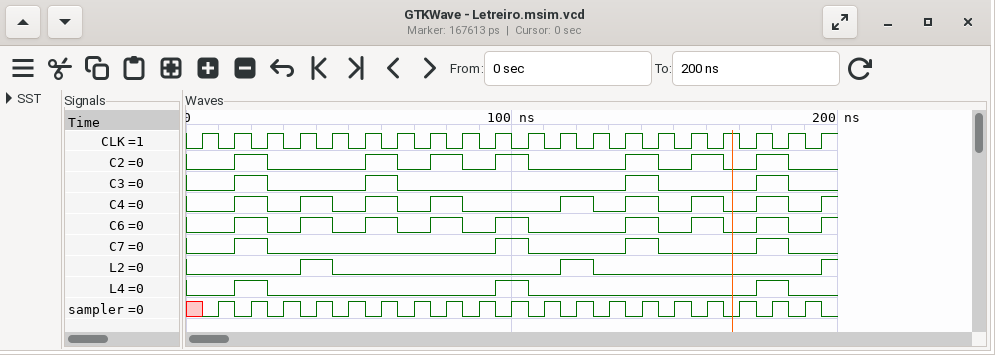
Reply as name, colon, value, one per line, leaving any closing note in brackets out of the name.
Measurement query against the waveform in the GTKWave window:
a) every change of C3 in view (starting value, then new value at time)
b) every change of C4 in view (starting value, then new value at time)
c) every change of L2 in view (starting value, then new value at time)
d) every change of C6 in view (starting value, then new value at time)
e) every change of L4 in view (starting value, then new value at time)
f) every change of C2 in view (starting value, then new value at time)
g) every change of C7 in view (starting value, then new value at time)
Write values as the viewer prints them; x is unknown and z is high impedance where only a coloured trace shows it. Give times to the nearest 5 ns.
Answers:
every change of C3 in view: 0, 1 at 15 ns, 0 at 25 ns, 1 at 55 ns, 0 at 65 ns, 1 at 135 ns, 0 at 145 ns, 1 at 175 ns, 0 at 185 ns
every change of C4 in view: 0, 1 at 15 ns, 0 at 25 ns, 1 at 35 ns, 0 at 45 ns, 1 at 55 ns, 0 at 65 ns, 1 at 75 ns, 0 at 85 ns, 1 at 115 ns, 0 at 125 ns, 1 at 135 ns, 0 at 145 ns, 1 at 155 ns, 0 at 165 ns, 1 at 175 ns, 0 at 185 ns, 1 at 195 ns
every change of L2 in view: 0, 1 at 35 ns, 0 at 45 ns, 1 at 115 ns, 0 at 125 ns, 1 at 195 ns
every change of C6 in view: 0, 1 at 15 ns, 0 at 25 ns, 1 at 35 ns, 0 at 45 ns, 1 at 55 ns, 0 at 65 ns, 1 at 75 ns, 0 at 85 ns, 1 at 95 ns, 0 at 105 ns, 1 at 135 ns, 0 at 145 ns, 1 at 155 ns, 0 at 165 ns, 1 at 175 ns, 0 at 185 ns, 1 at 195 ns
every change of L4 in view: 0, 1 at 15 ns, 0 at 25 ns, 1 at 95 ns, 0 at 105 ns, 1 at 175 ns, 0 at 185 ns
every change of C2 in view: 0, 1 at 15 ns, 0 at 25 ns, 1 at 55 ns, 0 at 65 ns, 1 at 75 ns, 0 at 85 ns, 1 at 95 ns, 0 at 105 ns, 1 at 135 ns, 0 at 145 ns, 1 at 155 ns, 0 at 165 ns, 1 at 175 ns, 0 at 185 ns
every change of C7 in view: 0, 1 at 15 ns, 0 at 25 ns, 1 at 95 ns, 0 at 105 ns, 1 at 135 ns, 0 at 145 ns, 1 at 175 ns, 0 at 185 ns
